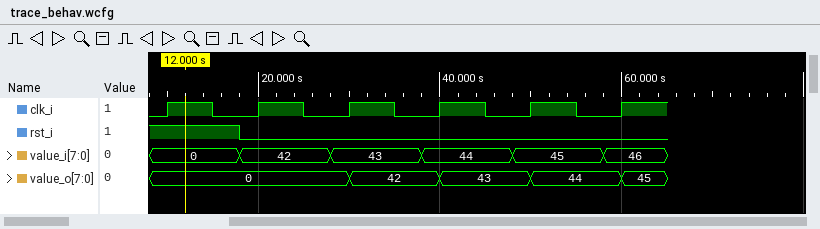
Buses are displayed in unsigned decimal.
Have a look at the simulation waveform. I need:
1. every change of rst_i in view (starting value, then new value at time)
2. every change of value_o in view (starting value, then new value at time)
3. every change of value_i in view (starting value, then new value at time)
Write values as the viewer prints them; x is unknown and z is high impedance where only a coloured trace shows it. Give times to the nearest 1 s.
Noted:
1, 0 at 18 s
0, 42 at 30 s, 43 at 40 s, 44 at 50 s, 45 at 60 s
0, 42 at 18 s, 43 at 28 s, 44 at 38 s, 45 at 48 s, 46 at 58 s
